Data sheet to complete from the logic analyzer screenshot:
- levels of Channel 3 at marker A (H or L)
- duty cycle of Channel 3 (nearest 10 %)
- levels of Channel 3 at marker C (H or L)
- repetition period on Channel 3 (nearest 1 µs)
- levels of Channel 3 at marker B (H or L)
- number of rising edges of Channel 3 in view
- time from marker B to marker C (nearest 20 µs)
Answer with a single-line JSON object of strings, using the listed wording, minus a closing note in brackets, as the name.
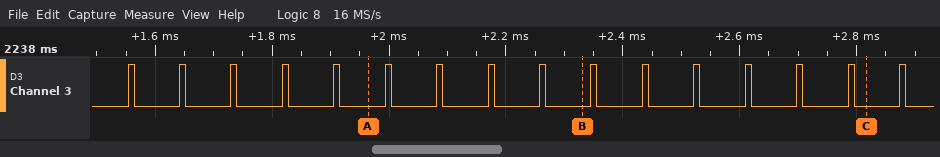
{"levels of Channel 3 at marker A": "Channel 3=L", "duty cycle of Channel 3": "10 %", "levels of Channel 3 at marker C": "Channel 3=L", "repetition period on Channel 3": "88 µs", "levels of Channel 3 at marker B": "Channel 3=L", "number of rising edges of Channel 3 in view": "16", "time from marker B to marker C": "480 µs"}
